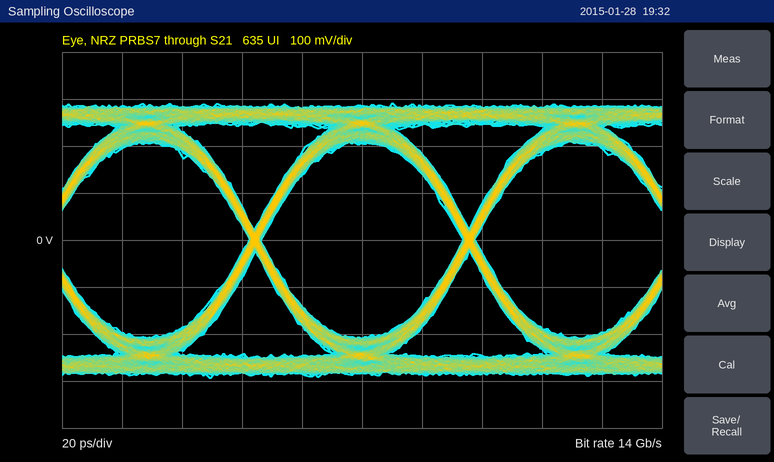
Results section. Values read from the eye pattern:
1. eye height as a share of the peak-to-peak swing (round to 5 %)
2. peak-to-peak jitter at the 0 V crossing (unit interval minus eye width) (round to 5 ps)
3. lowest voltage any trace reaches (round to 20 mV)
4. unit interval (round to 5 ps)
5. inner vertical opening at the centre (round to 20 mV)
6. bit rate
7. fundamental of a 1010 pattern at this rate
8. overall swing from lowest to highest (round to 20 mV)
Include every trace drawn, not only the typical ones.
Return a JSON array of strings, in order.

["70 %", "5 ps", "-300 mV", "70 ps", "420 mV", "14 Gb/s", "7 GHz", "580 mV"]
